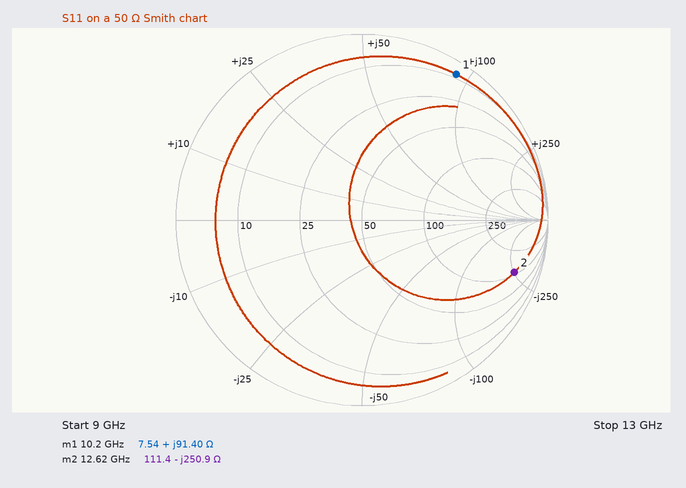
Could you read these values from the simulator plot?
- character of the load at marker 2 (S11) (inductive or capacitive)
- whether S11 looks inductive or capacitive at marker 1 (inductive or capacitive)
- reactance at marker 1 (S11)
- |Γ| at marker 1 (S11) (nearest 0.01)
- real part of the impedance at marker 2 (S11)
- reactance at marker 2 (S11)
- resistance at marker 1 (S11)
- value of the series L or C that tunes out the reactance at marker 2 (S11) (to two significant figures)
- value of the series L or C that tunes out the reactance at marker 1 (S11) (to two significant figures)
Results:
capacitive
inductive
+91.40 Ω
0.93
111.4 Ω
-250.9 Ω
7.54 Ω
3.2 nH
170 fF
